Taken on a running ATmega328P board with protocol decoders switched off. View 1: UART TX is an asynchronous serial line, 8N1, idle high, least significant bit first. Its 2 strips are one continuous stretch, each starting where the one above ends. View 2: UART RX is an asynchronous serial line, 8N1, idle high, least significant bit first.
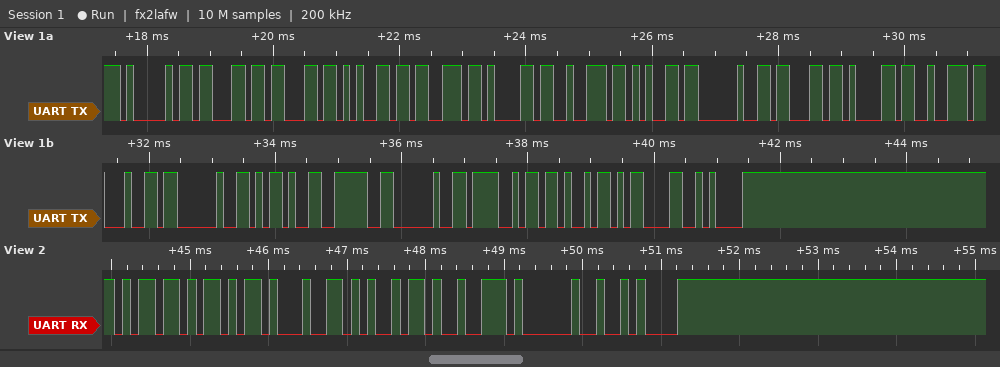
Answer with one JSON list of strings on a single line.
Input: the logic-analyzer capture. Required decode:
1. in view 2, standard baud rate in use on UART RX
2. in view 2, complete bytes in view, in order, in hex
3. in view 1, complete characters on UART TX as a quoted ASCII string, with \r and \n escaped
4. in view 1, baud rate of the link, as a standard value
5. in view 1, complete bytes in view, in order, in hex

["9600 baud", "6D 6B 64 69 72 20 0A", "\"Accesare card -> OK\\r\\n\"", "9600 baud", "41 63 63 65 73 61 72 65 20 63 61 72 64 20 2D 3E 20 4F 4B 0D 0A"]
